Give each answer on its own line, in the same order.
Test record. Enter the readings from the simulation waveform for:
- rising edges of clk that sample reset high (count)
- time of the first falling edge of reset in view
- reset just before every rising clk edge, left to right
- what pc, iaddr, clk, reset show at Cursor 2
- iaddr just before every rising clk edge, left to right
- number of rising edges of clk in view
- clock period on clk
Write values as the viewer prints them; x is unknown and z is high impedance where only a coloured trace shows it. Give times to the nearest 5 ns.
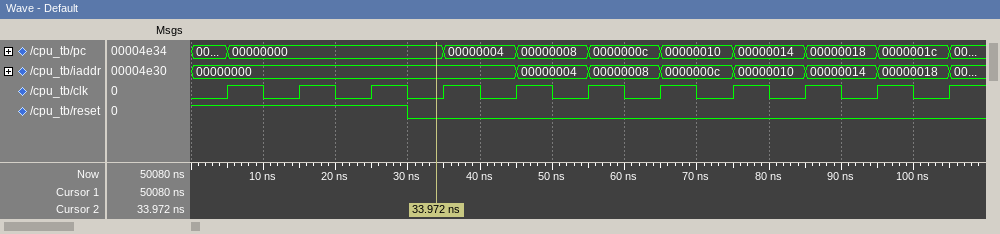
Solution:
3
30 ns
1 1 1 0 0 0 0 0 0 0 0
pc=00000000, iaddr=00000000, clk=0, reset=0
00000000, 00000000, 00000000, 00000000, 00000000, 00000004, 00000008, 0000000c, 00000010, 00000014, 00000018
11
10 ns
